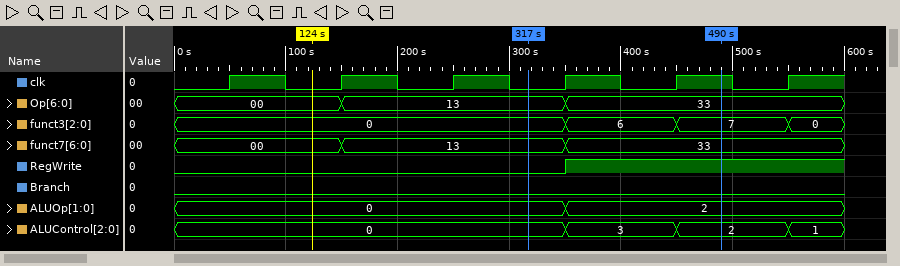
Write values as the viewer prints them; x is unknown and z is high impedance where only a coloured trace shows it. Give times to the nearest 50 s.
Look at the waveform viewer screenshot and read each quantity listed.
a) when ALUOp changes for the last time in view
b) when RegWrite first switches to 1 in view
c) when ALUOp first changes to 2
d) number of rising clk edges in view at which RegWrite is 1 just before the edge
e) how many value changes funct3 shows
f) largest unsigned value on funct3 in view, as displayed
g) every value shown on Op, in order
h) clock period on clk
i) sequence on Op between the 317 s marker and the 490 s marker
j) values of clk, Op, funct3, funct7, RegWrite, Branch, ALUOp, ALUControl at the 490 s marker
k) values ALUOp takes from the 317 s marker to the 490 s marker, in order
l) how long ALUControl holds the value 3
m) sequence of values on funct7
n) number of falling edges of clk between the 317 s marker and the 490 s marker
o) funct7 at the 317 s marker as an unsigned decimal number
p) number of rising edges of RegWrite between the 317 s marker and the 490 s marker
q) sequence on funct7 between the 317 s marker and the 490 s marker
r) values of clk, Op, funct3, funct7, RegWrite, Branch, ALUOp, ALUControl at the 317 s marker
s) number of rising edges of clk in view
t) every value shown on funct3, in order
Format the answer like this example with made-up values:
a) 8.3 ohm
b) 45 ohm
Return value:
a) 350 s
b) 350 s
c) 350 s
d) 2
e) 3
f) 7
g) 00, 13, 33
h) 100 s
i) 13, 33
j) clk=1, Op=33, funct3=7, funct7=33, RegWrite=1, Branch=0, ALUOp=2, ALUControl=2
k) 0, 2
l) 100 s
m) 00, 13, 33
n) 1
o) 19
p) 1
q) 13, 33
r) clk=0, Op=13, funct3=0, funct7=13, RegWrite=0, Branch=0, ALUOp=0, ALUControl=0
s) 6
t) 0, 6, 7, 0
